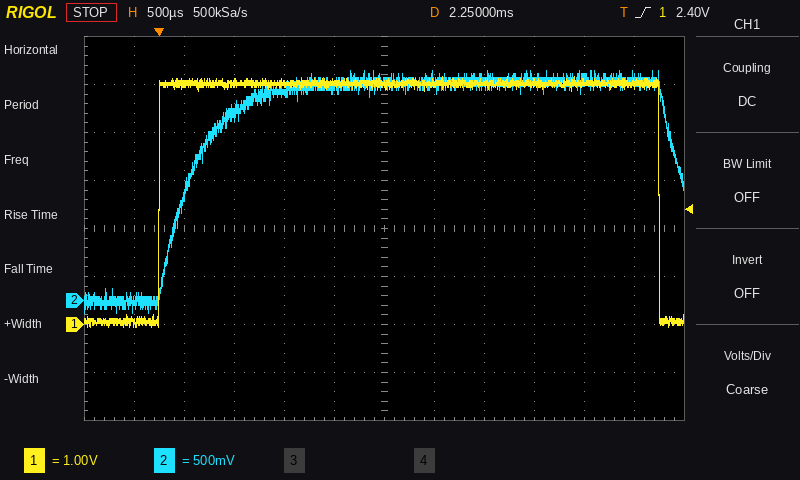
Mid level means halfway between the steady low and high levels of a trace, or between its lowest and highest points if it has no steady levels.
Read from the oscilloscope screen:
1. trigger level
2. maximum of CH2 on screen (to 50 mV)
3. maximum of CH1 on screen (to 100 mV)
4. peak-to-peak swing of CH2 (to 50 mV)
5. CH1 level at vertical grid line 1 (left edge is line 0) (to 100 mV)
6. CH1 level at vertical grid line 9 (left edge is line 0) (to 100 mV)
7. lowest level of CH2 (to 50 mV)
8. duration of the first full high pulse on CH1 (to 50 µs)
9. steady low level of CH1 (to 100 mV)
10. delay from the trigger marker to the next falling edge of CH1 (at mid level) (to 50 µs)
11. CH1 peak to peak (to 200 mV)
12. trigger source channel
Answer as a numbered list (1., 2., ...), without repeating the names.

1. 2.40 V
2. 2.40 V
3. 5.2 V
4. 2.50 V
5. 100 mV
6. 5.0 V
7. -100 mV
8. 5.00 ms
9. 100 mV
10. 5.00 ms
11. 5.2 V
12. CH1
